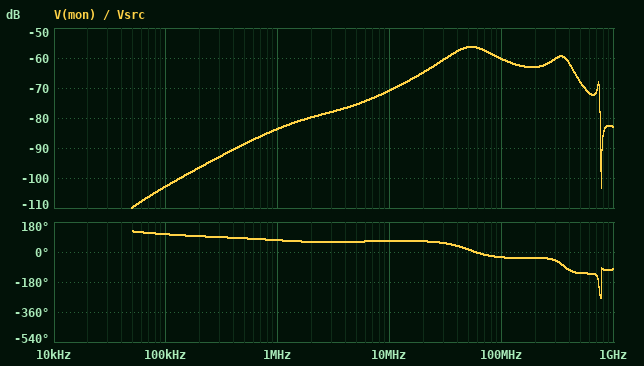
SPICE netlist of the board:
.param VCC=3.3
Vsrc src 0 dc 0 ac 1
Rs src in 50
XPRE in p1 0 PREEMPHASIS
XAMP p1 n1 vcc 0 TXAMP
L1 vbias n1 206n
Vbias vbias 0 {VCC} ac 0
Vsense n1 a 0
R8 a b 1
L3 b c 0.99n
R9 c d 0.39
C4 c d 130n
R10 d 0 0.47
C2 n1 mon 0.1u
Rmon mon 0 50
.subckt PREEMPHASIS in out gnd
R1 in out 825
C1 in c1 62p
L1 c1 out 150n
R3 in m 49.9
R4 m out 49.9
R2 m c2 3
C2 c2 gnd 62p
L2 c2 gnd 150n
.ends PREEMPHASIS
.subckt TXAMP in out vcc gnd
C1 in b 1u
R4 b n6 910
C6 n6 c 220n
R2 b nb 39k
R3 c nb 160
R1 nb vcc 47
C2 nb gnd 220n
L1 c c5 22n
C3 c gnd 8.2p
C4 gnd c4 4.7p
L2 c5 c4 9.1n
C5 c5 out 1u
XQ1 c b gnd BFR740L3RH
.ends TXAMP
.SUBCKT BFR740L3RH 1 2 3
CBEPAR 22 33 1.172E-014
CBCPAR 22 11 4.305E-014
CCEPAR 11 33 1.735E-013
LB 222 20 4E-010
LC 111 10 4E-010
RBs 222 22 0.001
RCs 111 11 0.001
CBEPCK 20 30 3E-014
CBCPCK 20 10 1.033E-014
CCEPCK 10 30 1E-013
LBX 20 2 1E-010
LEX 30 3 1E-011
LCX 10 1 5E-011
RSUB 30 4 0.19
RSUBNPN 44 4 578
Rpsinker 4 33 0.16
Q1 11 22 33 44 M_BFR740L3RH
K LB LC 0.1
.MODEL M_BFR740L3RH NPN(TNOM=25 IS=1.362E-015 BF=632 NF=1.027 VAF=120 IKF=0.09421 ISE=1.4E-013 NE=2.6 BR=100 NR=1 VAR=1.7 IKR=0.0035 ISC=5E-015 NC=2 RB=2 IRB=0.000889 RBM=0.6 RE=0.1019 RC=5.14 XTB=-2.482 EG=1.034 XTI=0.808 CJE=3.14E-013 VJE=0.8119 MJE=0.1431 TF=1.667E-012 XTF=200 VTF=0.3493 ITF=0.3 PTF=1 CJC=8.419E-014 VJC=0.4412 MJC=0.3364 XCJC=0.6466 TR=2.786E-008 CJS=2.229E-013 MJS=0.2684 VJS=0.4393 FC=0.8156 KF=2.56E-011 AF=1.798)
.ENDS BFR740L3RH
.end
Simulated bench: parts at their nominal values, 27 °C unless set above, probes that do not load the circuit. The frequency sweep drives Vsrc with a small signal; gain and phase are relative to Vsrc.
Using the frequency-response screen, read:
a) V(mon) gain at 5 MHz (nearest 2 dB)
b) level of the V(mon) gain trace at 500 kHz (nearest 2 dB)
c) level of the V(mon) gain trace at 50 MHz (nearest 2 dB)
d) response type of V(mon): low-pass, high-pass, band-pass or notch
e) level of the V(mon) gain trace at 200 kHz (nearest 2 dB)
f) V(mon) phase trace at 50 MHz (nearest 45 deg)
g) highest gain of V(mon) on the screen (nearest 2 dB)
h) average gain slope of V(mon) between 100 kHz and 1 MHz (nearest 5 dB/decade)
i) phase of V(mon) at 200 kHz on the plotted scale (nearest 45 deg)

-76 dB
-88 dB
-56 dB
band-pass
-96 dB
0 deg
-56 dB
20 dB/decade
90 deg
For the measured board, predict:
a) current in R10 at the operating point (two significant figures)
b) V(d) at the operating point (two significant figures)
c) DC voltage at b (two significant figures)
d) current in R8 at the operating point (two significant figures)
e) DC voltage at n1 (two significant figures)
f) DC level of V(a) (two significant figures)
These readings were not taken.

1.8 A
830 mV
1.5 V
1.8 A
3.3 V
3.3 V
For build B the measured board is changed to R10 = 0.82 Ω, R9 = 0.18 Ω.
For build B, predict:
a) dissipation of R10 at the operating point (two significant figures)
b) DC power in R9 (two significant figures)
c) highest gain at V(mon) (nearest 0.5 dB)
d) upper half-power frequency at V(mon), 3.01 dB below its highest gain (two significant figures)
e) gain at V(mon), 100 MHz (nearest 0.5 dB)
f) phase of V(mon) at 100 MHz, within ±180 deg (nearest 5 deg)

2.2 W
490 mW
-54.5 dB
86 MHz
-59.0 dB
-35 deg
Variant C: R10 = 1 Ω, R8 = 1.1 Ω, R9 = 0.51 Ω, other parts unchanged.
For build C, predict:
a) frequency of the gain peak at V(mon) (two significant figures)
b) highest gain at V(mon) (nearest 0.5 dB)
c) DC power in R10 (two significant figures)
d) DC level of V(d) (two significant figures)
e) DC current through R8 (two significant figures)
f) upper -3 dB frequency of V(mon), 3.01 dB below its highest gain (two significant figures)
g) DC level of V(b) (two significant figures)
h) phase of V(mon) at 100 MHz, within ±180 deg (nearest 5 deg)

53 MHz
-53.5 dB
1.6 W
1.3 V
1.3 A
86 MHz
1.9 V
-40 deg
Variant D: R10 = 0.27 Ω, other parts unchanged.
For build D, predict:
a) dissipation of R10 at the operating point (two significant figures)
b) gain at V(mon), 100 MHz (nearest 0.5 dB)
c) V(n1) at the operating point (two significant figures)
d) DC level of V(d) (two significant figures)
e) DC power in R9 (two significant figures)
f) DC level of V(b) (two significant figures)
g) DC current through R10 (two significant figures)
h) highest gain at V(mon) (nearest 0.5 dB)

1.1 W
-61.5 dB
3.3 V
540 mV
1.5 W
1.3 V
2.0 A
-57.5 dB
